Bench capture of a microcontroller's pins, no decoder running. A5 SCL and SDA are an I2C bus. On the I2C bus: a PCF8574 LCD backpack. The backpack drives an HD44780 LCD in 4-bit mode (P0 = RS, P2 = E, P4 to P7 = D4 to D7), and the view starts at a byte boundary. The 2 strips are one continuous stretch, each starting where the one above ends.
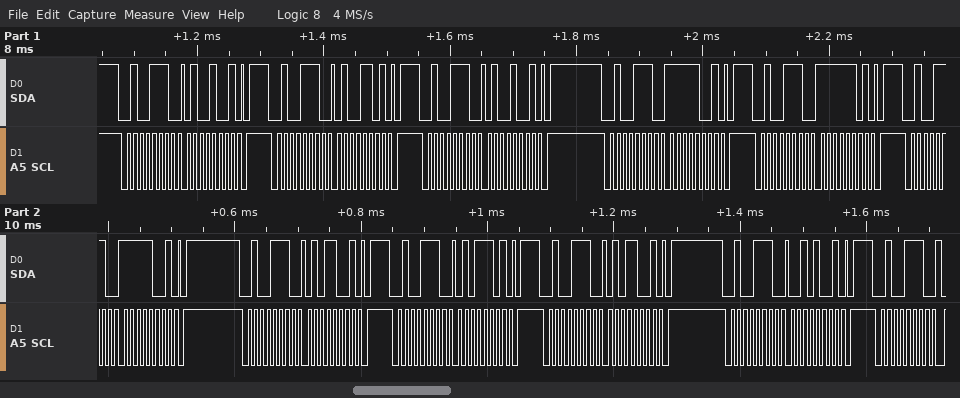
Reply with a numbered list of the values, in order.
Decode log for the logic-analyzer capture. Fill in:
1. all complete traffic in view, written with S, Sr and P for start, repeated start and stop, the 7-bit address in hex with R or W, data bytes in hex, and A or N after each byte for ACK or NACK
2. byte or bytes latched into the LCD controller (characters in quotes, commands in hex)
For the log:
1. S 27W A 49 A P S 27W A 4D A P S 27W A 49 A P S 27W A F9 A P S 27W A FD A P S 27W A F9 A P S 27W A 59 A P S 27W A 5D A P S 27W A 59 A P S 27W A 29 A P S 27W A
2. 'O'
